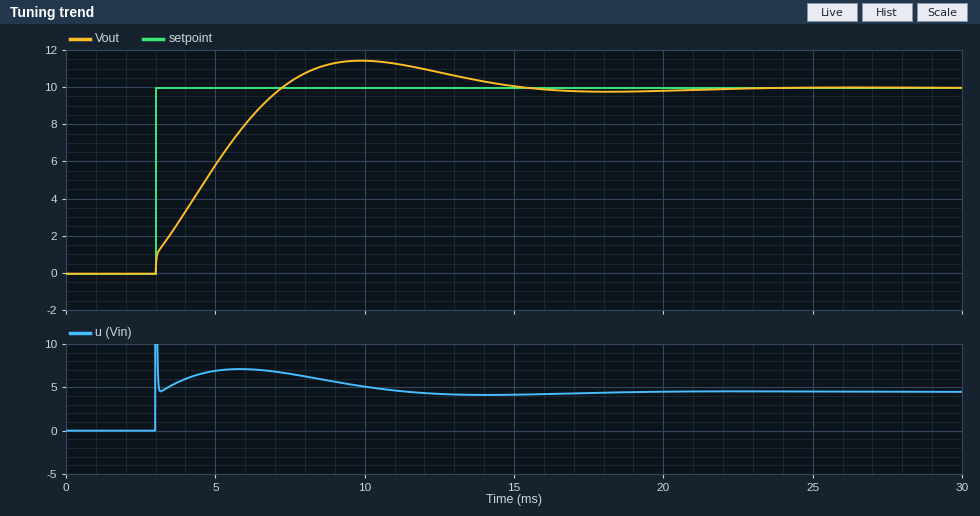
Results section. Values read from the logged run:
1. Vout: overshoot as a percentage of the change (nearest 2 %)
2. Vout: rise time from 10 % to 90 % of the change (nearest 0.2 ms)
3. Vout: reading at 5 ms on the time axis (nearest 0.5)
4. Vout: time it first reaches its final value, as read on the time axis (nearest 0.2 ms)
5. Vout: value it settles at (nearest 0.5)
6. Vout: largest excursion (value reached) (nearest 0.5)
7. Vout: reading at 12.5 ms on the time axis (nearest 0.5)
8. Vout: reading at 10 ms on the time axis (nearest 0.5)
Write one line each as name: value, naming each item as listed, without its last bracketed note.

Vout: overshoot as a percentage of the change: 14 %
Vout: rise time from 10 % to 90 % of the change: 3.4 ms
Vout: reading at 5 ms on the time axis: 6.0
Vout: time it first reaches its final value, as read on the time axis: 7.2 ms
Vout: value it settles at: 10.0
Vout: largest excursion (value reached): 11.5
Vout: reading at 12.5 ms on the time axis: 11.0
Vout: reading at 10 ms on the time axis: 11.5
